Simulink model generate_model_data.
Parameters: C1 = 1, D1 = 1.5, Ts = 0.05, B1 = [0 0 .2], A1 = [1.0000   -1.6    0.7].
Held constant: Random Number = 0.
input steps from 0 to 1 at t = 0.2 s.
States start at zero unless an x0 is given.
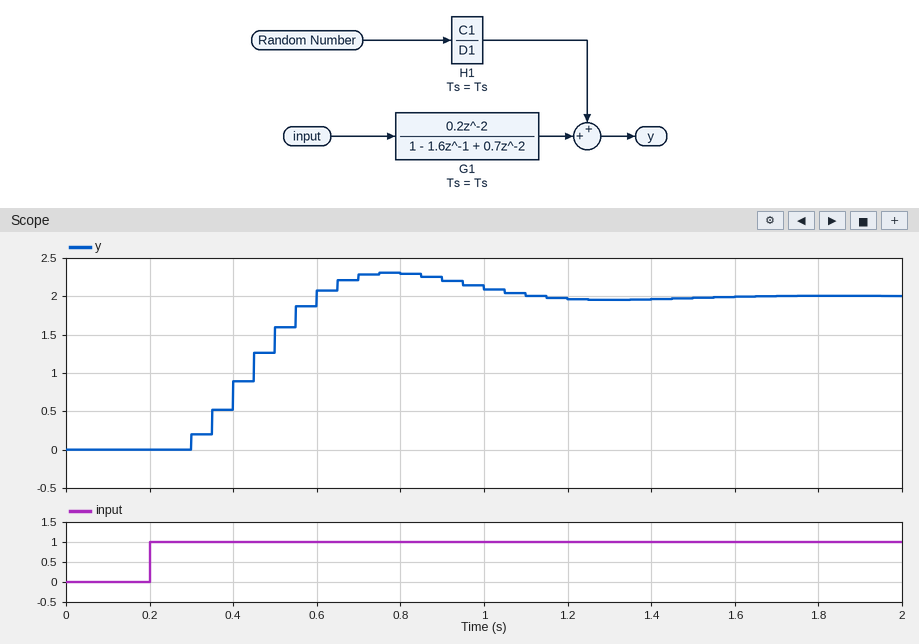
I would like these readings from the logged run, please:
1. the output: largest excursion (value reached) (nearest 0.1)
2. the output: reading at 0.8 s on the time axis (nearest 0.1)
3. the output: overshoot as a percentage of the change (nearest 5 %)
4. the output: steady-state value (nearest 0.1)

2.3
2.3
15 %
2.0
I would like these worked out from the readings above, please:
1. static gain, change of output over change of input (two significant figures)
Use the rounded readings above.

2.0
